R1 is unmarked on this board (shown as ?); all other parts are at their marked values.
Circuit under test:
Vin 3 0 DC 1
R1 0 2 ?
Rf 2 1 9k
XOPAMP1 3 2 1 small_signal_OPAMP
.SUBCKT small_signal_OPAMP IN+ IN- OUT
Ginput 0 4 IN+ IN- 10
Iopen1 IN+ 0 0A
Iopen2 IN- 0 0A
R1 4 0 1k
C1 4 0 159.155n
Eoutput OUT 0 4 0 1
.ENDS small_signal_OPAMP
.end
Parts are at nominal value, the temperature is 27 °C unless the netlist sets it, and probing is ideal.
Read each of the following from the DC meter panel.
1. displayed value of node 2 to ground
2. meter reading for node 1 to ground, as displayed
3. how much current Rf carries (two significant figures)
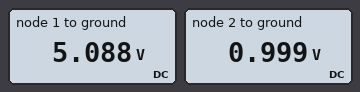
0.999 V
5.088 V
450 µA
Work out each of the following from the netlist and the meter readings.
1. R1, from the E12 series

2.2 kΩ
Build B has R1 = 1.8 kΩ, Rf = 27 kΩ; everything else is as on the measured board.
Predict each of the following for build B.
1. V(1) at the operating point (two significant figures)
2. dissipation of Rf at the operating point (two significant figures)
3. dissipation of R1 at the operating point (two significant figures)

16 V
8.3 mW
550 µW
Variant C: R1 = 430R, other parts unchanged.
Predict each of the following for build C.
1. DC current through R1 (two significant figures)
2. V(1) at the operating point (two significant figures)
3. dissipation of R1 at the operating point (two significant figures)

2.3 mA
22 V
2.3 mW
